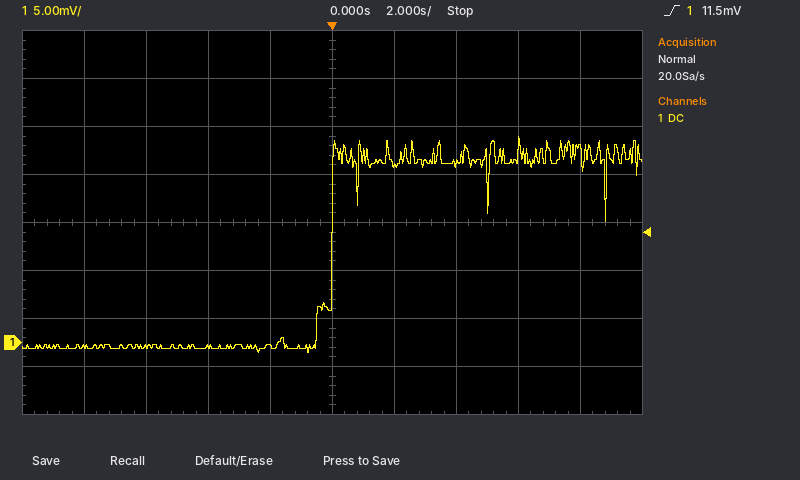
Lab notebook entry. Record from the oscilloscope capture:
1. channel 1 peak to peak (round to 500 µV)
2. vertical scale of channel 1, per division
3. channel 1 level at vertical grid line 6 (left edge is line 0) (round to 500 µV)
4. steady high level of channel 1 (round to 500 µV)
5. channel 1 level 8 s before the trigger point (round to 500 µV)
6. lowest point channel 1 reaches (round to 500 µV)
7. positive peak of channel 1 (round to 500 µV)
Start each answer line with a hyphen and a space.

- 22.5 mV
- 5 mV
- 18.5 mV
- 18.5 mV
- -500 µV
- -1.0 mV
- 21.5 mV
